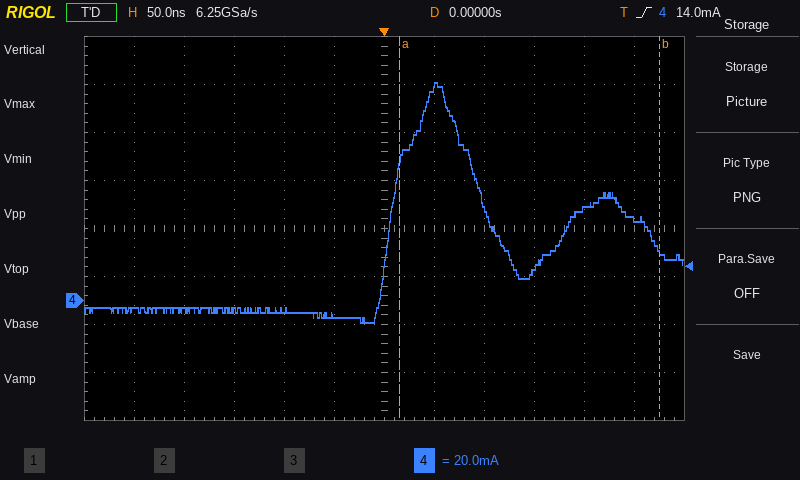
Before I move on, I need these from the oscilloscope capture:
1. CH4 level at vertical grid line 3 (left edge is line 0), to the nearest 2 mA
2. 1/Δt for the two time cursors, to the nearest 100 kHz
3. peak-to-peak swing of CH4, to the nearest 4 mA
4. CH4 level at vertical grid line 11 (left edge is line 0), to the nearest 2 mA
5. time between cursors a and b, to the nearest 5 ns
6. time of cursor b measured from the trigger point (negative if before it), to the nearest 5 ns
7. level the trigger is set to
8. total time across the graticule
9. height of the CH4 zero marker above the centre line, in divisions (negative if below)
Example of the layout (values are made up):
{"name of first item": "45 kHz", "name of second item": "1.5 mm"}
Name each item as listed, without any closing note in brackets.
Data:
{"CH4 level at vertical grid line 3 (left edge is line 0), to the nearest 2 mA": "-4 mA", "1/Δt for the two time cursors, to the nearest 100 kHz": "3.8 MHz", "peak-to-peak swing of CH4, to the nearest 4 mA": "100 mA", "CH4 level at vertical grid line 11 (left edge is line 0), to the nearest 2 mA": "34 mA", "time between cursors a and b, to the nearest 5 ns": "260 ns", "time of cursor b measured from the trigger point (negative if before it), to the nearest 5 ns": "+275 ns", "level the trigger is set to": "14.0 mA", "total time across the graticule": "600 ns", "height of the CH4 zero marker above the centre line, in divisions": "-1.5 div"}
